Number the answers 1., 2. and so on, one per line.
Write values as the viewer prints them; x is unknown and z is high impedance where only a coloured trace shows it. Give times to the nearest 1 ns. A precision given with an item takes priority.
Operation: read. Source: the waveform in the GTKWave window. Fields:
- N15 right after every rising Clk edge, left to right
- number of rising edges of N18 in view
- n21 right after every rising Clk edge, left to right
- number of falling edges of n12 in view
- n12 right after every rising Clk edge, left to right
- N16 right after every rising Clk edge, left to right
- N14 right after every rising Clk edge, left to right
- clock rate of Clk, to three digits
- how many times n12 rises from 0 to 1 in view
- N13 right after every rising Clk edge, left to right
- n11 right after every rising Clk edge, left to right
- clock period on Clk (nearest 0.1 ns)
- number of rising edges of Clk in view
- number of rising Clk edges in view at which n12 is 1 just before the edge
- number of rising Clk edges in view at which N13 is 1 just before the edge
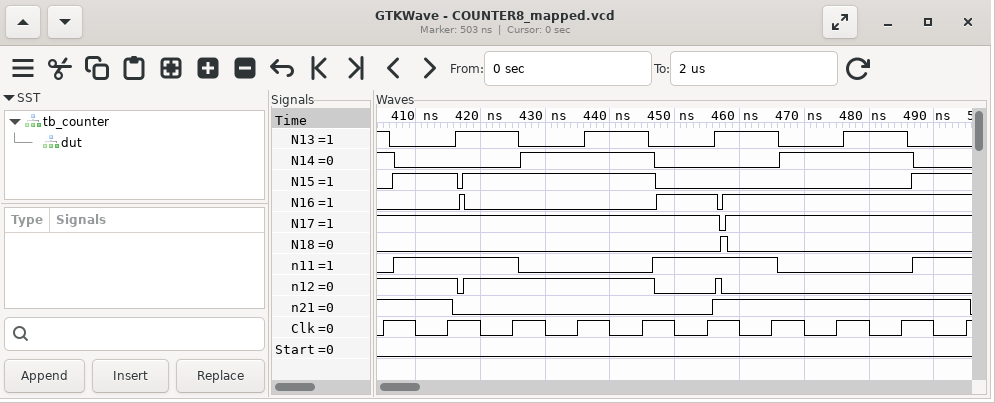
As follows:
1. 0 1 1 1 1 0 0 0 0 1
2. 1
3. 1 1 0 0 0 0 1 1 1 1
4. 3
5. 1 1 1 1 1 0 0 0 0 0
6. 0 0 0 0 0 1 1 1 1 1
7. 1 0 0 1 1 0 0 1 1 0
8. 100 MHz
9. 2
10. 1 0 1 0 1 0 1 0 1 0
11. 0 1 1 0 0 1 1 0 0 1
12. 10 ns
13. 10
14. 5
15. 5
